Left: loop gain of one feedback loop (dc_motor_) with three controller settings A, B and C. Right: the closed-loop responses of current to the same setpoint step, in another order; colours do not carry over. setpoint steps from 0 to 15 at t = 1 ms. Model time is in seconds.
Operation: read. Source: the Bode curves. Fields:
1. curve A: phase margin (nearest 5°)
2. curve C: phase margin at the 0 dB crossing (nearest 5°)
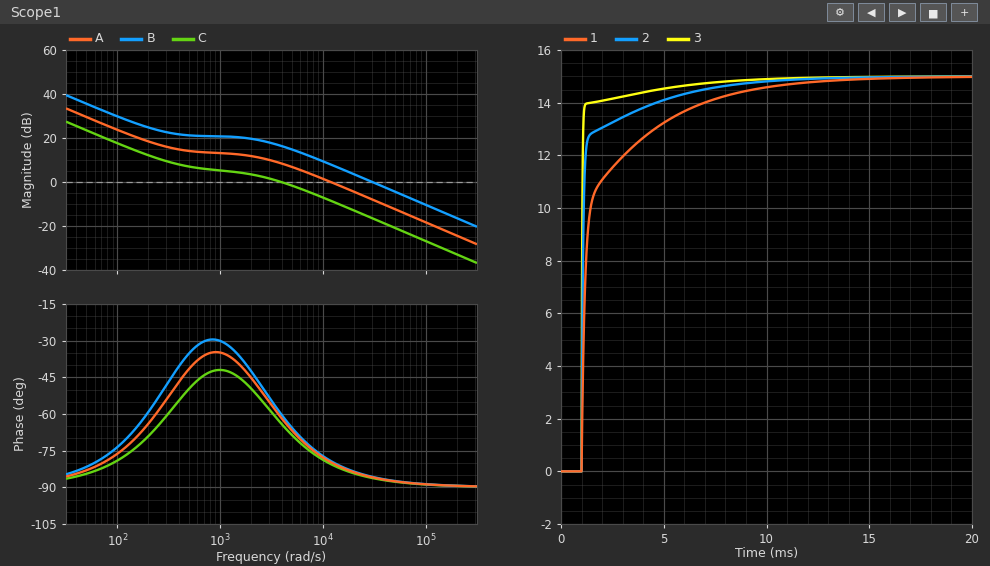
100°
115°
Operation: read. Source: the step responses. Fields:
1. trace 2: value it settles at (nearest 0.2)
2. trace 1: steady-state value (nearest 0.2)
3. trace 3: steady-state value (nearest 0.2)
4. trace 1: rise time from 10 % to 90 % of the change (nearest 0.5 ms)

15.0
15.0
15.0
4.5 ms
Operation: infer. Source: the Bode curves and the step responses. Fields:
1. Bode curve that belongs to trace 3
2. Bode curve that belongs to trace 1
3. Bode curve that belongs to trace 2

B
C
A
